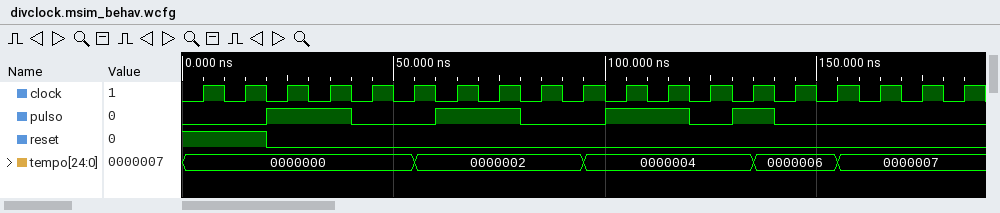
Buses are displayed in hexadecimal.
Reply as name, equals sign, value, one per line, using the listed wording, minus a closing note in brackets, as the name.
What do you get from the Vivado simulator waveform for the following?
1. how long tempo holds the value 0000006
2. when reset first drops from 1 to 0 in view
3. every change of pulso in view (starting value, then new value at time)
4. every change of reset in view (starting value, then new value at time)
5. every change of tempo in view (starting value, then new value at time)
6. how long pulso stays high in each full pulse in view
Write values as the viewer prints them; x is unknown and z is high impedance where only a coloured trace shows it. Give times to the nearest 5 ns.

how long tempo holds the value 0000006 = 20 ns
when reset first drops from 1 to 0 in view = 20 ns
every change of pulso in view = 0, 1 at 20 ns, 0 at 40 ns, 1 at 60 ns, 0 at 80 ns, 1 at 100 ns, 0 at 120 ns, 1 at 130 ns, 0 at 140 ns
every change of reset in view = 1, 0 at 20 ns
every change of tempo in view = 0000000, 0000002 at 55 ns, 0000004 at 95 ns, 0000006 at 135 ns, 0000007 at 155 ns
how long pulso stays high in each full pulse in view = 20 ns, 20 ns, 20 ns, 10 ns
